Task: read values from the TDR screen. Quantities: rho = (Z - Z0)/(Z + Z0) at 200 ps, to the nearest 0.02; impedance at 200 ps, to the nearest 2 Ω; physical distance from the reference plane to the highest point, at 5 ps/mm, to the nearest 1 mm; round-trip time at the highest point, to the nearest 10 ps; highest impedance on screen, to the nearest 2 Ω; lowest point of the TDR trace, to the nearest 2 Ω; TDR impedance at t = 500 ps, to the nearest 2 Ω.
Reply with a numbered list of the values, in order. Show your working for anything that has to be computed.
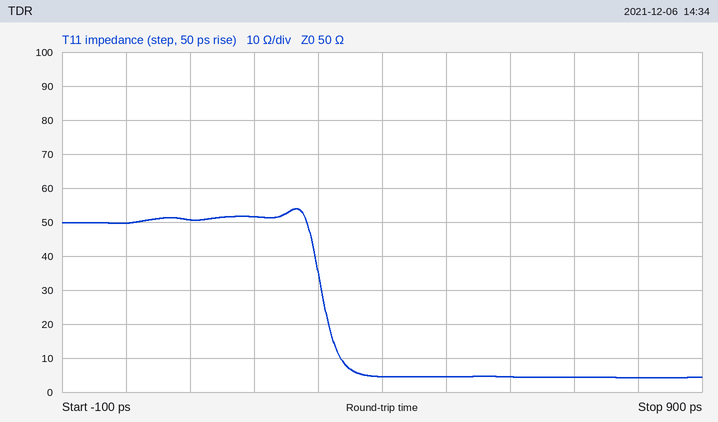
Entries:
1. (52 − 50)/(52 + 50) ≈ +0.02
2. 52 Ω
3. 270 ps / 2 / 5 ps/mm ≈ 27 mm
4. 270 ps
5. 54 Ω
6. 4 Ω
7. 4 Ω
